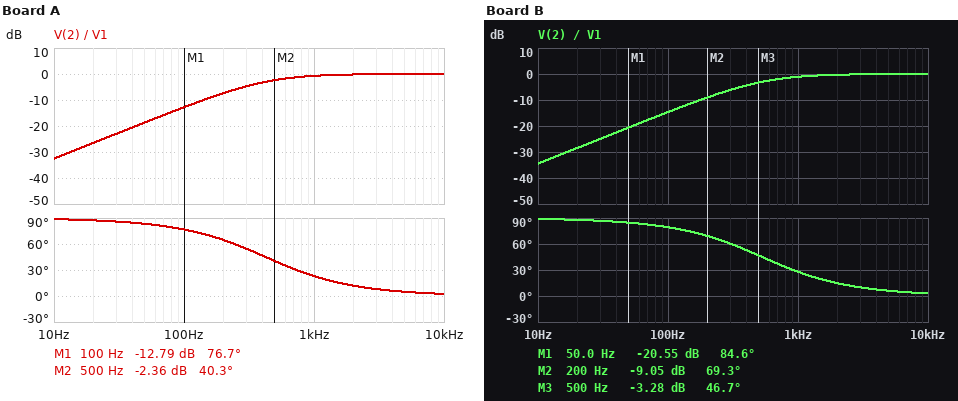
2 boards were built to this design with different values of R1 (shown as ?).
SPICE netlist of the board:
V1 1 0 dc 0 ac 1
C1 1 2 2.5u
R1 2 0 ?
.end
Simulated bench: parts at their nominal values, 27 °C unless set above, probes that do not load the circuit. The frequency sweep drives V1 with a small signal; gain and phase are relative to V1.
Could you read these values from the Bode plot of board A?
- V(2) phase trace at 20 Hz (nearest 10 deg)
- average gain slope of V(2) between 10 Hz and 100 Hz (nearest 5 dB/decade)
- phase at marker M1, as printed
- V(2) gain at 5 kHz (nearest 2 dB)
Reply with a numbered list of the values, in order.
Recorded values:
1. 90 deg
2. 20 dB/decade
3. 76.7 deg
4. 0 dB
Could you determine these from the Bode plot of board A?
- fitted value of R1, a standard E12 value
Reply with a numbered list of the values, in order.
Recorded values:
1. 150 Ω
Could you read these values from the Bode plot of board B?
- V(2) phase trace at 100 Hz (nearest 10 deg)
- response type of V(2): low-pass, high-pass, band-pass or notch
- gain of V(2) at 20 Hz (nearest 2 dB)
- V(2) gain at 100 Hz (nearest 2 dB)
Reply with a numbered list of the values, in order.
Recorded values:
1. 80 deg
2. high-pass
3. -28 dB
4. -14 dB
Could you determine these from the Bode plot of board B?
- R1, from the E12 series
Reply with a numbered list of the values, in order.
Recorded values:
1. 120 Ω
